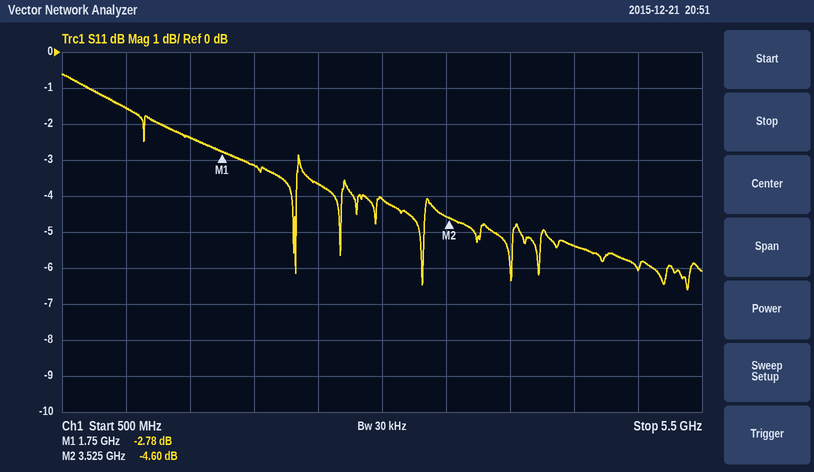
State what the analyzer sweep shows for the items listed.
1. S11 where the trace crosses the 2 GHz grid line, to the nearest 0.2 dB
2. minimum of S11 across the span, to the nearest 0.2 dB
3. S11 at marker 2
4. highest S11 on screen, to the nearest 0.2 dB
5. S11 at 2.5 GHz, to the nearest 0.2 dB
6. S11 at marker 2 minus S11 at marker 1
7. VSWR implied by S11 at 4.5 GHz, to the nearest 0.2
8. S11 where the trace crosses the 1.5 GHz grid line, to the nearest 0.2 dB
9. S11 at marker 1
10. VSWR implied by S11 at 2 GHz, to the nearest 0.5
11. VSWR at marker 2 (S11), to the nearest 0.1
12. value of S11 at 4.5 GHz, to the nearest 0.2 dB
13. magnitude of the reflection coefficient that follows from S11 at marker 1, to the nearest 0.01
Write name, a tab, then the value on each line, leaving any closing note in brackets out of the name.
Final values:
S11 where the trace crosses the 2 GHz grid line, to the nearest 0.2 dB	-3.2 dB
minimum of S11 across the span, to the nearest 0.2 dB	-6.6 dB
S11 at marker 2	-4.60 dB
highest S11 on screen, to the nearest 0.2 dB	-0.6 dB
S11 at 2.5 GHz, to the nearest 0.2 dB	-3.6 dB
S11 at marker 2 minus S11 at marker 1	-1.82 dB
VSWR implied by S11 at 4.5 GHz, to the nearest 0.2	3.4
S11 where the trace crosses the 1.5 GHz grid line, to the nearest 0.2 dB	-2.4 dB
S11 at marker 1	-2.78 dB
VSWR implied by S11 at 2 GHz, to the nearest 0.5	5.5
VSWR at marker 2 (S11), to the nearest 0.1	3.9
value of S11 at 4.5 GHz, to the nearest 0.2 dB	-5.4 dB
magnitude of the reflection coefficient that follows from S11 at marker 1, to the nearest 0.01	0.73
